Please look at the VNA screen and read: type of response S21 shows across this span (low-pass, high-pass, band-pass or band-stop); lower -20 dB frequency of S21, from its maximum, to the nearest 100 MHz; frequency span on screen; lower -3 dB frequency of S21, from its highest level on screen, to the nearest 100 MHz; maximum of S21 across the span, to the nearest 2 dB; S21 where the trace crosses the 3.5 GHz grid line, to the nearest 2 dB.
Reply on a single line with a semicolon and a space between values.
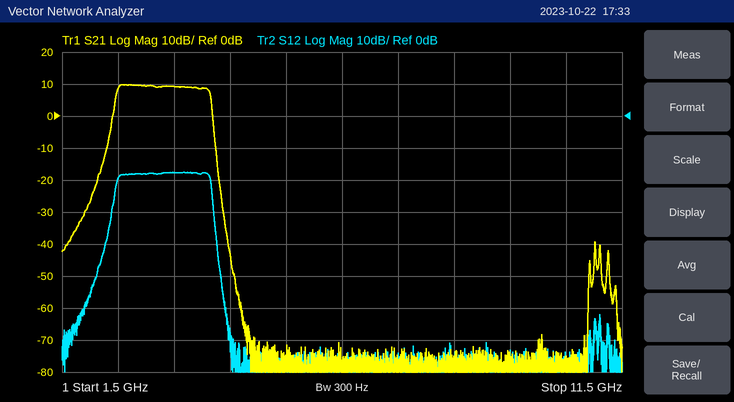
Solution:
band-pass; 2.3 GHz; 10 GHz; 2.5 GHz; 10 dB; 10 dB
